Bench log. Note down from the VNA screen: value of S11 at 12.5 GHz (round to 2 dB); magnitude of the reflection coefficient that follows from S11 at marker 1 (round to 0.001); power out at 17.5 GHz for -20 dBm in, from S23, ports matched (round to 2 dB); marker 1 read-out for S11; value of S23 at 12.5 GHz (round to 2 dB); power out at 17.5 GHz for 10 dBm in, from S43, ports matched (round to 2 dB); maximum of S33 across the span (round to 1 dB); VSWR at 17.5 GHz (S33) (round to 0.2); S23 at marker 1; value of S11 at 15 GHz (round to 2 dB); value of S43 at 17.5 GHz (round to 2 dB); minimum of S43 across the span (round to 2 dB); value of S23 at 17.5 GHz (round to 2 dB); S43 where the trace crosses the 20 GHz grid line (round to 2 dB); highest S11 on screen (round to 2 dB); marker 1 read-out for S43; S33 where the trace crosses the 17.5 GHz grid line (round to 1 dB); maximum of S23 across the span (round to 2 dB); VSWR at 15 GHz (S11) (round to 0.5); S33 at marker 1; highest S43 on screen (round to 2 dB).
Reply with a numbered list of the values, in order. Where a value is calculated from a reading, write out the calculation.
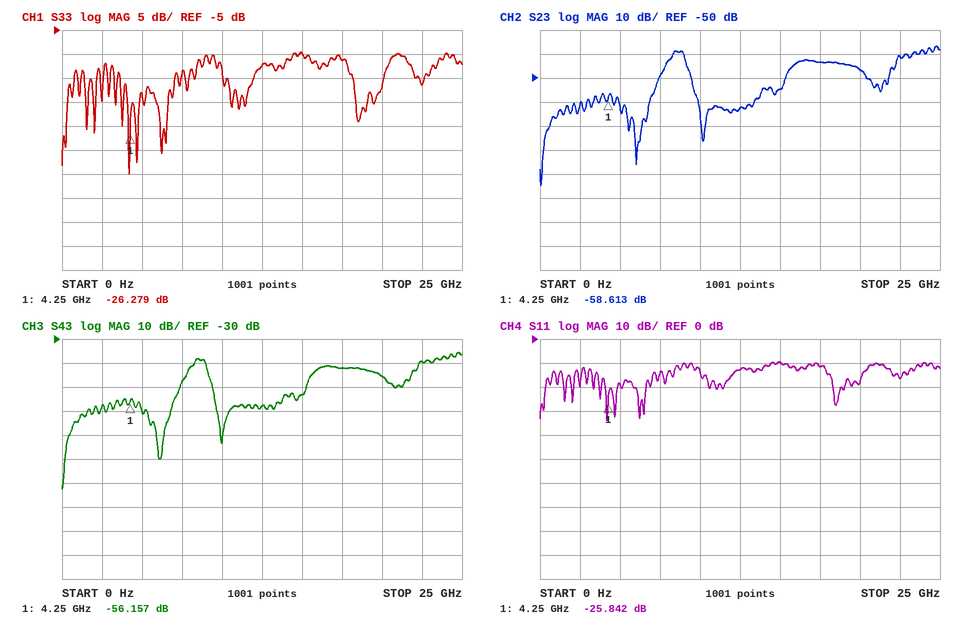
1. -12 dB
2. 10^(-25.842/20) ≈ 0.051
3. -20 dBm + (-44 dB) = -64 dBm
4. -25.842 dB
5. -62 dB
6. 10 dBm + (-42 dB) = -32 dBm
7. -10 dB
8. |Γ| = 10^(-11/20) = 0.2818; VSWR = (1 + 0.2818)/(1 − 0.2818) ≈ 1.8
9. -58.613 dB
10. -10 dB
11. -42 dB
12. -92 dB
13. -44 dB
14. -46 dB
15. -10 dB
16. -56.157 dB
17. -11 dB
18. -36 dB
19. |Γ| = 10^(-10/20) = 0.3162; VSWR = (1 + 0.3162)/(1 − 0.3162) ≈ 1.92, so 2.0 to the nearest 0.5
20. -26.279 dB
21. -36 dB
